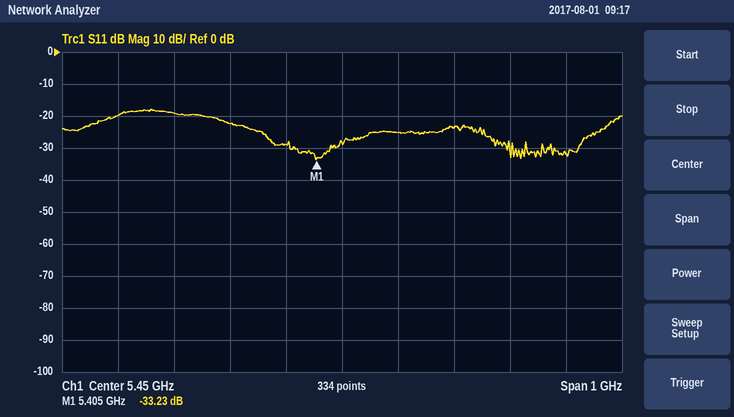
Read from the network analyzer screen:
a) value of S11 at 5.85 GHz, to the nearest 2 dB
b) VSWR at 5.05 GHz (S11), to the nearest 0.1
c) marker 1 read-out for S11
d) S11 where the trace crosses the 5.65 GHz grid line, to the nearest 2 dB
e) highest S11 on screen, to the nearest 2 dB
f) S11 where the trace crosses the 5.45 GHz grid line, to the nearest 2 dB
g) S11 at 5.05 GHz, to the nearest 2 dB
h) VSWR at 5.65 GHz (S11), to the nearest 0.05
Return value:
-32 dB
1.2
-33.23 dB
-24 dB
-18 dB
-28 dB
-20 dB
1.15
